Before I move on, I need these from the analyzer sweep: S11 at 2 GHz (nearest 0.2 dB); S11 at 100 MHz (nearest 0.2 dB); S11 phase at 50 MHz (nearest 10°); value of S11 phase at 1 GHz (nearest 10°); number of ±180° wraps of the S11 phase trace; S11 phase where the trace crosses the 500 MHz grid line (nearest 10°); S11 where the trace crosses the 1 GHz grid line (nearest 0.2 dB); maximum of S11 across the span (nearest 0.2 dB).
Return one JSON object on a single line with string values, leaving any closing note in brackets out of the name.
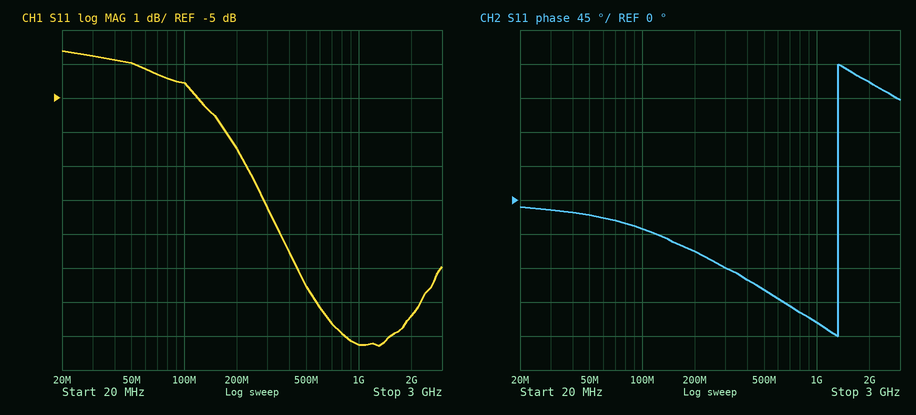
{"S11 at 2 GHz": "-11.4 dB", "S11 at 100 MHz": "-4.6 dB", "S11 phase at 50 MHz": "-20°", "value of S11 phase at 1 GHz": "-160°", "number of ±180° wraps of the S11 phase trace": "1", "S11 phase where the trace crosses the 500 MHz grid line": "-120°", "S11 where the trace crosses the 1 GHz grid line": "-12.2 dB", "maximum of S11 across the span": "-3.6 dB"}
